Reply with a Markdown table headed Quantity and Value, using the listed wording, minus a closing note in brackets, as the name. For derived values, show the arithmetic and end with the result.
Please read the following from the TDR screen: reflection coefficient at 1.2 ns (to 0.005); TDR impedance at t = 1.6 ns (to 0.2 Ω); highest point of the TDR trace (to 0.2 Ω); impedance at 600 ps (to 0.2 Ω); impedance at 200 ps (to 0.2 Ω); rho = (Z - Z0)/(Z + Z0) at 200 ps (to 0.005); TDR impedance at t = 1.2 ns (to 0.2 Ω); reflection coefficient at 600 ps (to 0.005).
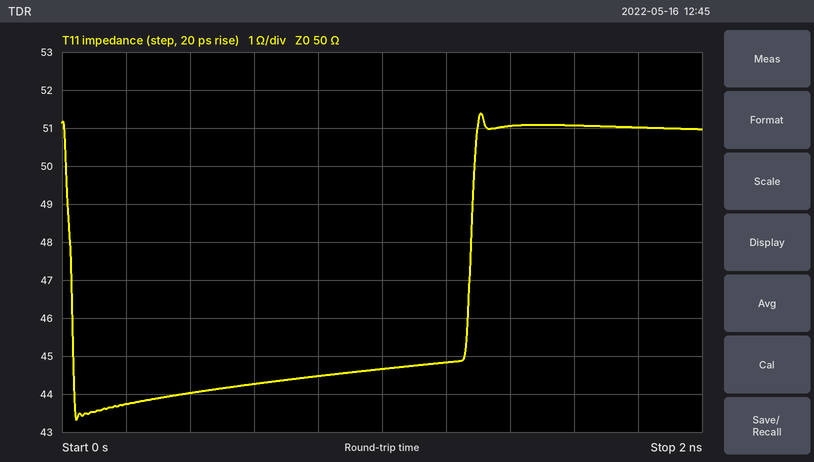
| Quantity | Value |
|---|---|
| reflection coefficient at 1.2 ns | (44.8 − 50)/(44.8 + 50) ≈ -0.055 |
| TDR impedance at t = 1.6 ns | 51.0 Ω |
| highest point of the TDR trace | 51.4 Ω |
| impedance at 600 ps | 44.2 Ω |
| impedance at 200 ps | 43.8 Ω |
| rho = (Z - Z0)/(Z + Z0) at 200 ps | (43.8 − 50)/(43.8 + 50) ≈ -0.0661, so -0.065 to the nearest 0.005 |
| TDR impedance at t = 1.2 ns | 44.8 Ω |
| reflection coefficient at 600 ps | (44.2 − 50)/(44.2 + 50) ≈ -0.0616, so -0.060 to the nearest 0.005 |
